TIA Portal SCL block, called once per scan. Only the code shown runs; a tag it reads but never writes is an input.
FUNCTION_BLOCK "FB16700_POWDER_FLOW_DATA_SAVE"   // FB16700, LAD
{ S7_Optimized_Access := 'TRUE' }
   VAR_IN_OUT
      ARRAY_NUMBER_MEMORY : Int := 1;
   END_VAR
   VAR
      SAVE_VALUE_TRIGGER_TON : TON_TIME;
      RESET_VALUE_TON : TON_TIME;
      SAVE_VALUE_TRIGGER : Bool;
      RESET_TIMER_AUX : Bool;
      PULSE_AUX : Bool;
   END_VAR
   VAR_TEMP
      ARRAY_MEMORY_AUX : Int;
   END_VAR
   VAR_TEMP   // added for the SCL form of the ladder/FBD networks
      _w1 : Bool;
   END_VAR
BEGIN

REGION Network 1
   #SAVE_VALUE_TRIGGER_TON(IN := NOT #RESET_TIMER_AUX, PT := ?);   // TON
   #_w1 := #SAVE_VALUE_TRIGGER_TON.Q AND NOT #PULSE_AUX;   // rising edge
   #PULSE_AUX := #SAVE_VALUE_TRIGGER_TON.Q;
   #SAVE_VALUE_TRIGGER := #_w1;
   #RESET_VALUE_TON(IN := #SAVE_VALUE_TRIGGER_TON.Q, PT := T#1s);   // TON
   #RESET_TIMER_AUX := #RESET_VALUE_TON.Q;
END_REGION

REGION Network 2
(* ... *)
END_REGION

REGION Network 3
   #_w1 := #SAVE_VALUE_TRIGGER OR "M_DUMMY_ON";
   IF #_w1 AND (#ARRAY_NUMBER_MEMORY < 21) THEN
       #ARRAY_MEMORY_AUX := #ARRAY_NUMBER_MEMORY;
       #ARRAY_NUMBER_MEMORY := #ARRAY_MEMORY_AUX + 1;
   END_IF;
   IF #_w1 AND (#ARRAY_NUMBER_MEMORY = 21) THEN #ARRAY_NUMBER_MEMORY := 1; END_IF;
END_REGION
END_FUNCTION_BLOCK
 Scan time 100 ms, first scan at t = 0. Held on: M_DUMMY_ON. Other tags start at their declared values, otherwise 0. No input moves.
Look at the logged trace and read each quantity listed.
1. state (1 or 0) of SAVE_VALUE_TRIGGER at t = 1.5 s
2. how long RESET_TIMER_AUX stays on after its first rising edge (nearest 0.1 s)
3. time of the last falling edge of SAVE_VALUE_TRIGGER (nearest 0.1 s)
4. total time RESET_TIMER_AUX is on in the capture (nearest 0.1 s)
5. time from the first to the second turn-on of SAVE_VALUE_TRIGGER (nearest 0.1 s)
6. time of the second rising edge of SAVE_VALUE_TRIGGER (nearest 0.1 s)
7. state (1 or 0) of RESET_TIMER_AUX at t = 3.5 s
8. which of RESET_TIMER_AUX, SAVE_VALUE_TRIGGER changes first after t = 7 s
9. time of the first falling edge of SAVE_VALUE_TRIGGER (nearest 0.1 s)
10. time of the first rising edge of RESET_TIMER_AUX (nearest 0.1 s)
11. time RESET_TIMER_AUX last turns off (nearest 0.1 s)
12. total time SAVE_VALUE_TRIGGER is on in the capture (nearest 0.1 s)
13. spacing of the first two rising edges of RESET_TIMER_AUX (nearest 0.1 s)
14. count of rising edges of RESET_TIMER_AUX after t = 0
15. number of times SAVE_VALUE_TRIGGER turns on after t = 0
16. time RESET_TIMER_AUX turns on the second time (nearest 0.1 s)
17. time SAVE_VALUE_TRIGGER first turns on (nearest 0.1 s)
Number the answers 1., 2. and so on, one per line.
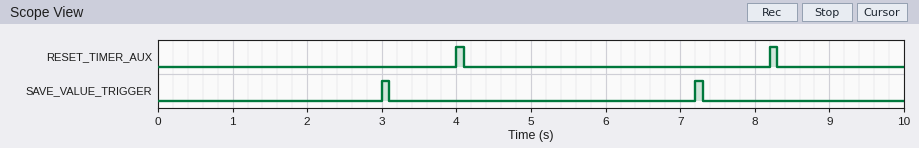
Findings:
1. 0
2. 0.1 s
3. 7.3 s
4. 0.2 s
5. 4.2 s
6. 7.2 s
7. 0
8. SAVE_VALUE_TRIGGER
9. 3.1 s
10. 4.0 s
11. 8.3 s
12. 0.2 s
13. 4.2 s
14. 2
15. 2
16. 8.2 s
17. 3.0 s
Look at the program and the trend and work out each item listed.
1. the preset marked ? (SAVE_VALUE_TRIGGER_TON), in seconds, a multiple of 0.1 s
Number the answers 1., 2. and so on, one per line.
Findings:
1. 3.0 s
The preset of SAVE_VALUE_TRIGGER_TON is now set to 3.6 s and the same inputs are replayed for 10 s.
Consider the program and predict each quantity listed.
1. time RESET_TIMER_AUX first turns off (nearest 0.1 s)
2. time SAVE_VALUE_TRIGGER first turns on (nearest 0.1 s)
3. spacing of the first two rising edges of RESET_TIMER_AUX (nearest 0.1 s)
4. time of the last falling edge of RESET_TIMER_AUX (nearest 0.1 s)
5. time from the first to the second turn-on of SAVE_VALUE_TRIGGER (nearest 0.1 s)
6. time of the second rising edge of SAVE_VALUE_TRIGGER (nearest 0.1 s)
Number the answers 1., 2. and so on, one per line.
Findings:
1. 4.7 s
2. 3.6 s
3. 4.8 s
4. 9.5 s
5. 4.8 s
6. 8.4 s
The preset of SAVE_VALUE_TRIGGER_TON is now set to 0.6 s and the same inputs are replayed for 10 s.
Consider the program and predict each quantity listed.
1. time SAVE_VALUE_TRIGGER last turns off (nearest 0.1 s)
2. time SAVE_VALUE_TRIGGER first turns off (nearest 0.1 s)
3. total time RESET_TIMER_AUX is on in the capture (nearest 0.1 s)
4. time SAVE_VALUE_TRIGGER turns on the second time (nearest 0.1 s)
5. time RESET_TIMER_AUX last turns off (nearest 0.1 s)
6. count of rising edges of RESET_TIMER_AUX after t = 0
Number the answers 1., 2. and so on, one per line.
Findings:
1. 9.7 s
2. 0.7 s
3. 0.5 s
4. 2.4 s
5. 8.9 s
6. 5
